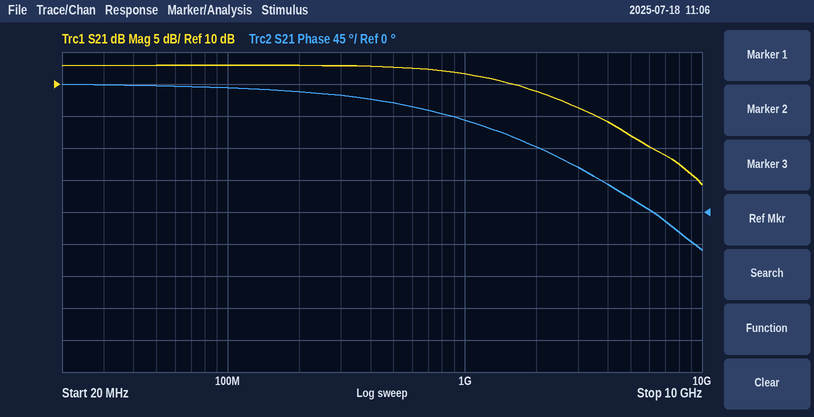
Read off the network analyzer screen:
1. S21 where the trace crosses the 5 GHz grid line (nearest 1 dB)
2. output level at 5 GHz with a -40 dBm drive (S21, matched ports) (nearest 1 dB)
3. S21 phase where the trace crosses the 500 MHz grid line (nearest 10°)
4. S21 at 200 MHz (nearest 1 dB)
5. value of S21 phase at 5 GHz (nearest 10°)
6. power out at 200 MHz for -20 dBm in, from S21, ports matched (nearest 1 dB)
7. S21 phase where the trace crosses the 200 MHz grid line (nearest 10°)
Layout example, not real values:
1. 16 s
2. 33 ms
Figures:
1. 2 dB
2. -38 dBm
3. 150°
4. 13 dB
5. 20°
6. -7 dBm
7. 170°
